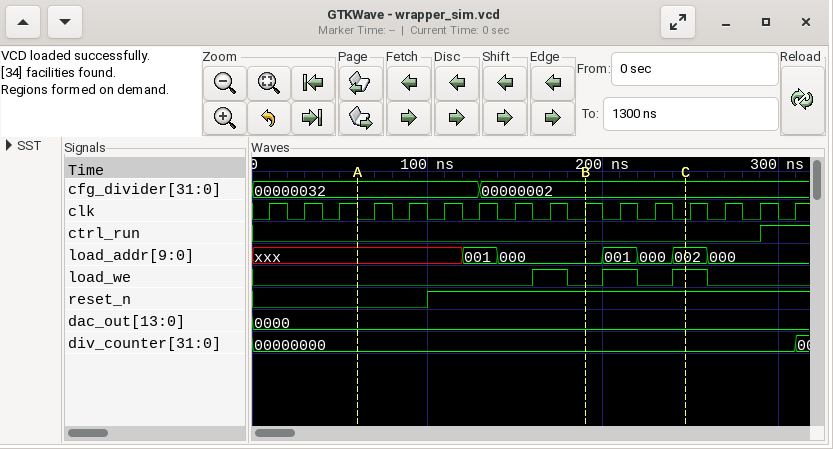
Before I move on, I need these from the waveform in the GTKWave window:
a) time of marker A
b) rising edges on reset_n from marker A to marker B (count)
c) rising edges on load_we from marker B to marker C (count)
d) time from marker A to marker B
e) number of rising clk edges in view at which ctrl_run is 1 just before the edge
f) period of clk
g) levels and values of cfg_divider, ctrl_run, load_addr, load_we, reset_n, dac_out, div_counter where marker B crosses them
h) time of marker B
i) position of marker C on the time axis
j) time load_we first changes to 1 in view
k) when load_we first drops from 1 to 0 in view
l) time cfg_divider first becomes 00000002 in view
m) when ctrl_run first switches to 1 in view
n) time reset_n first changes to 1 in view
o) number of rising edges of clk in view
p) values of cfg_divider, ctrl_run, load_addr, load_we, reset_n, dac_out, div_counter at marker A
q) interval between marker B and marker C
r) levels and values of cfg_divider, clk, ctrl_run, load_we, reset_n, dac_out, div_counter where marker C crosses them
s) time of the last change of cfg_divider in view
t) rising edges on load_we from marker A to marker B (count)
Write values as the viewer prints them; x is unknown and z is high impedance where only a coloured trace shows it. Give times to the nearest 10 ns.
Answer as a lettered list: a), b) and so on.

a) 60 ns
b) 1
c) 2
d) 130 ns
e) 1
f) 20 ns
g) cfg_divider=00000002, ctrl_run=0, load_addr=000, load_we=0, reset_n=1, dac_out=0000, div_counter=00000000
h) 190 ns
i) 250 ns
j) 160 ns
k) 180 ns
l) 130 ns
m) 290 ns
n) 100 ns
o) 16
p) cfg_divider=00000032, ctrl_run=0, load_addr=xxx, load_we=0, reset_n=0, dac_out=0000, div_counter=00000000
q) 60 ns
r) cfg_divider=00000002, clk=0, ctrl_run=0, load_we=1, reset_n=1, dac_out=0000, div_counter=00000000
s) 130 ns
t) 1
